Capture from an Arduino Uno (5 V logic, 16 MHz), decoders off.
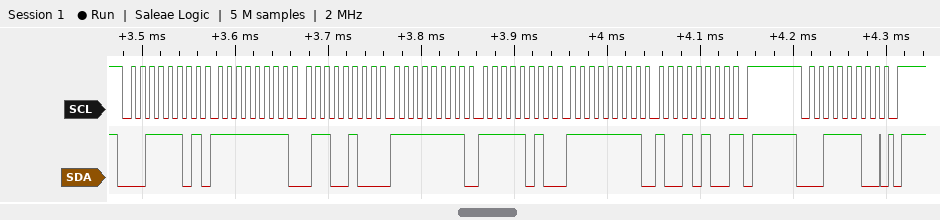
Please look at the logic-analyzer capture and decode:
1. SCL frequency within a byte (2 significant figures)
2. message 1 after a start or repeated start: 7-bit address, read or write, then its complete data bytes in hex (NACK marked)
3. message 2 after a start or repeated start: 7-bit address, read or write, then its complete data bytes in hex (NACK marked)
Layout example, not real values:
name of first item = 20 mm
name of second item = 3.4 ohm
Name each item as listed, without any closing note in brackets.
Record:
SCL frequency within a byte = 100 kHz
message 1 after a start or repeated start: 7-bit address, read or write, then its complete data bytes in hex = 0x1E read: FF 64 FF FA FF 94 NACK
message 2 after a start or repeated start: 7-bit address, read or write, then its complete data bytes in hex = 0x1E write
